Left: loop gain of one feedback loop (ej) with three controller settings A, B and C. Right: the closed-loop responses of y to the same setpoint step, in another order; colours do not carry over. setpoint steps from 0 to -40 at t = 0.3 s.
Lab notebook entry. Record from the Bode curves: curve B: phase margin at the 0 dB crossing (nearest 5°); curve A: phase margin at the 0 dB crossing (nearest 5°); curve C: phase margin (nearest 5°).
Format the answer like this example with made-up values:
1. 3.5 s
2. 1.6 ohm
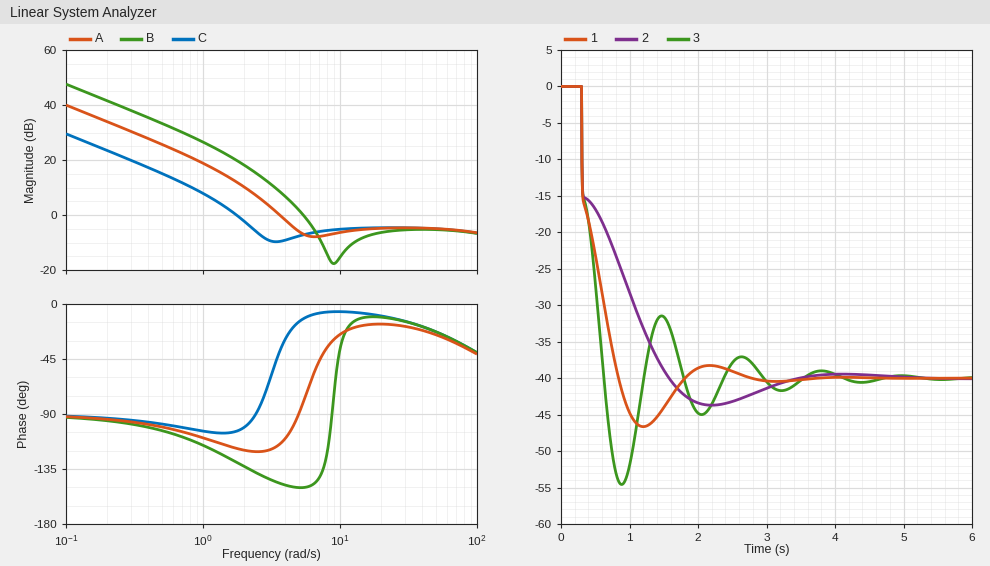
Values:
1. 30°
2. 65°
3. 75°
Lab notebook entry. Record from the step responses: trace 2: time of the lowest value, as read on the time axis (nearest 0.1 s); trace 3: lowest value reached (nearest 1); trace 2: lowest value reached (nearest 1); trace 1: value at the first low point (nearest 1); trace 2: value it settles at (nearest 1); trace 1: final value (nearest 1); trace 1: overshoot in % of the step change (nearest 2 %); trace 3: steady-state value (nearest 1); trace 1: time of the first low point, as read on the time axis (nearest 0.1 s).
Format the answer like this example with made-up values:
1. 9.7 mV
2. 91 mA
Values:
1. 2.2 s
2. -55
3. -44
4. -47
5. -40
6. -40
7. 16 %
8. -40
9. 1.2 s
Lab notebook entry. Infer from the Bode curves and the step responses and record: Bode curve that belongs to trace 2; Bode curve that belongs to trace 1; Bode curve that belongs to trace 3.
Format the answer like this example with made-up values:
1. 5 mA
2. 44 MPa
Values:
1. C
2. A
3. B
